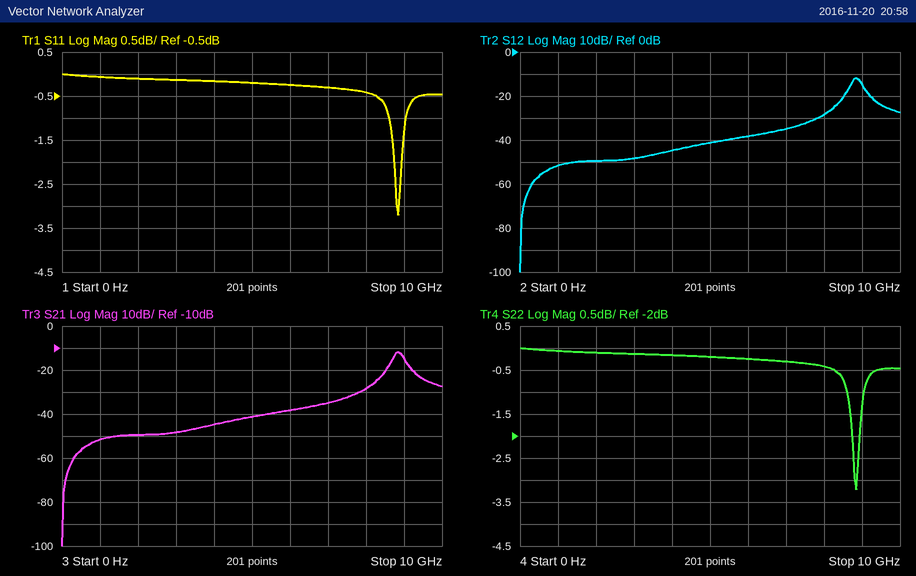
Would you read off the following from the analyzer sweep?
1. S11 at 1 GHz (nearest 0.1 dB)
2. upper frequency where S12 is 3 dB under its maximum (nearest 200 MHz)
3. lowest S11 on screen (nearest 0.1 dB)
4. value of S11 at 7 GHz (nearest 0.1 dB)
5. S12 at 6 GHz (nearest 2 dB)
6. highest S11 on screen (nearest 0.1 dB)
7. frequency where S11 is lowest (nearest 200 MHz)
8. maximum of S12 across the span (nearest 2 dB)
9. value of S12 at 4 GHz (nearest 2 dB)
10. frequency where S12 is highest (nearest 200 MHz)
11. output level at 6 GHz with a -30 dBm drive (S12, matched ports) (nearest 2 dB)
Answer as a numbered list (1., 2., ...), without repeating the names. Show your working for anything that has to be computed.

1. -0.1 dB
2. 9.0 GHz
3. -3.2 dB
4. -0.3 dB
5. -38 dB
6. 0.0 dB
7. 8.8 GHz
8. -12 dB
9. -44 dB
10. 8.8 GHz
11. -30 dBm + (-38 dB) = -68 dBm
